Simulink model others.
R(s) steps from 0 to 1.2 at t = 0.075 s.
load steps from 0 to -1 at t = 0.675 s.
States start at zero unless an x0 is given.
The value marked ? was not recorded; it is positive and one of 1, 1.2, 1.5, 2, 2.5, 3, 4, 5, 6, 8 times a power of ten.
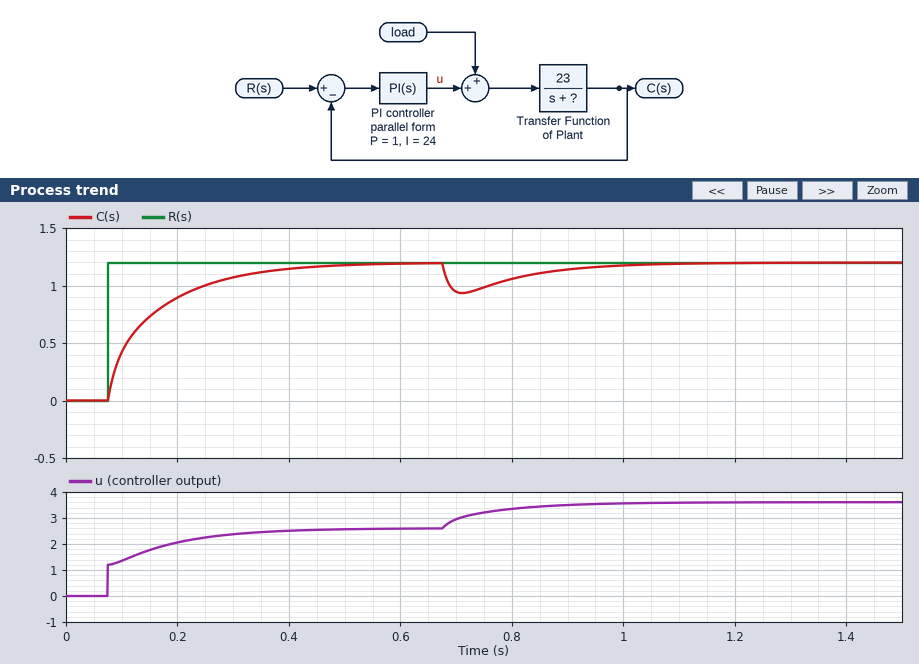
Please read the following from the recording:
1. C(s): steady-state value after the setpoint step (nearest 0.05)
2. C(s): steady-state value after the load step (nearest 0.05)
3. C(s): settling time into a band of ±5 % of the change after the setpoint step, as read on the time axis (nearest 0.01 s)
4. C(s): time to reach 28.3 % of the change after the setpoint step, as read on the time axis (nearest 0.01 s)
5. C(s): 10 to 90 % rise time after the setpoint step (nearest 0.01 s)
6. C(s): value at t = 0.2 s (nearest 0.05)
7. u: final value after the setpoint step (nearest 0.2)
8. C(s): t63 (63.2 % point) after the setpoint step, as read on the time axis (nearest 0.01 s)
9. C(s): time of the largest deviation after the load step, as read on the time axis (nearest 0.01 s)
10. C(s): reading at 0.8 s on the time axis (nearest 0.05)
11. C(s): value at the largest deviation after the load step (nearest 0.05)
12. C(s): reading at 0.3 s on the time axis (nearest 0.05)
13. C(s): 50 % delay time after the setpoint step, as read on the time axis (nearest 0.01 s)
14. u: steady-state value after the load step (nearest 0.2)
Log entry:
1.20
1.20
0.39 s
0.09 s
0.23 s
0.90
2.6
0.16 s
0.71 s
1.05
0.95
1.05
0.12 s
3.6
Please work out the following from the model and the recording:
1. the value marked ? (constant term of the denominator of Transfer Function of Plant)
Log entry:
50
